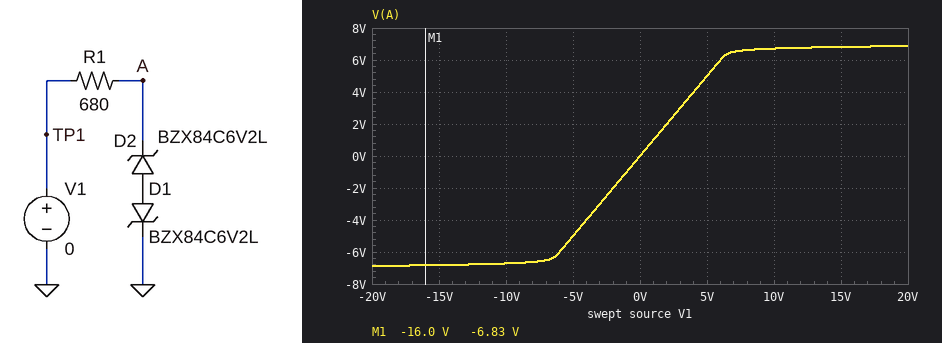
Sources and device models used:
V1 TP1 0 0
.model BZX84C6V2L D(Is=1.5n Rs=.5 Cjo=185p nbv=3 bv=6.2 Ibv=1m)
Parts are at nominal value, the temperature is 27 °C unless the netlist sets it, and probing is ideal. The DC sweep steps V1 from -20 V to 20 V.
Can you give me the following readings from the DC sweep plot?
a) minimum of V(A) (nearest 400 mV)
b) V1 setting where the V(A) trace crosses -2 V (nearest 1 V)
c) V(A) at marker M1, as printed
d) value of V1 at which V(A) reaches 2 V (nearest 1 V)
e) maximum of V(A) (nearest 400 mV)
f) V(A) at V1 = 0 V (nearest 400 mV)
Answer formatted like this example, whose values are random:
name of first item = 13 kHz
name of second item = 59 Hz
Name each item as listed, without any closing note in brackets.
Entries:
minimum of V(A) = -6.8 V
V1 setting where the V(A) trace crosses -2 V = -2 V
V(A) at marker M1, as printed = -6.83 V
value of V1 at which V(A) reaches 2 V = 2 V
maximum of V(A) = 6.8 V
V(A) at V1 = 0 V = 0 V
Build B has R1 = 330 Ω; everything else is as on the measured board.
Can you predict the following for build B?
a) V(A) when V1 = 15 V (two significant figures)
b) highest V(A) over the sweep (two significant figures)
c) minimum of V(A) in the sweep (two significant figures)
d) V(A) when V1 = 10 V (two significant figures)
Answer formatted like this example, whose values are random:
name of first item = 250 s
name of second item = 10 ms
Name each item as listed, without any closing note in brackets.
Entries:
V(A) when V1 = 15 V = 6.9 V
highest V(A) over the sweep = 7.0 V
minimum of V(A) in the sweep = -7.0 V
V(A) when V1 = 10 V = 6.8 V
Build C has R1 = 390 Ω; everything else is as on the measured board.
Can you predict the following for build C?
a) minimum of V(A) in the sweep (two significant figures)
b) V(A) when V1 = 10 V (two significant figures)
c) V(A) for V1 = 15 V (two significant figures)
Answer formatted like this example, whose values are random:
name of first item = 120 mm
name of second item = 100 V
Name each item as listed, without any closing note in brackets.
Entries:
minimum of V(A) in the sweep = -6.9 V
V(A) when V1 = 10 V = 6.8 V
V(A) for V1 = 15 V = 6.9 V
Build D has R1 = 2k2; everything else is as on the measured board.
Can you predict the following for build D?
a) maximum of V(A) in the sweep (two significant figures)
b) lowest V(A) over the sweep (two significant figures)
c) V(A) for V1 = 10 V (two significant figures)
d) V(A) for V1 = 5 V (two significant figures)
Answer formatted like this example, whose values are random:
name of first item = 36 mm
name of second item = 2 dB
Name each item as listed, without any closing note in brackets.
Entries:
maximum of V(A) in the sweep = 6.7 V
lowest V(A) over the sweep = -6.7 V
V(A) for V1 = 10 V = 6.6 V
V(A) for V1 = 5 V = 5.0 V
